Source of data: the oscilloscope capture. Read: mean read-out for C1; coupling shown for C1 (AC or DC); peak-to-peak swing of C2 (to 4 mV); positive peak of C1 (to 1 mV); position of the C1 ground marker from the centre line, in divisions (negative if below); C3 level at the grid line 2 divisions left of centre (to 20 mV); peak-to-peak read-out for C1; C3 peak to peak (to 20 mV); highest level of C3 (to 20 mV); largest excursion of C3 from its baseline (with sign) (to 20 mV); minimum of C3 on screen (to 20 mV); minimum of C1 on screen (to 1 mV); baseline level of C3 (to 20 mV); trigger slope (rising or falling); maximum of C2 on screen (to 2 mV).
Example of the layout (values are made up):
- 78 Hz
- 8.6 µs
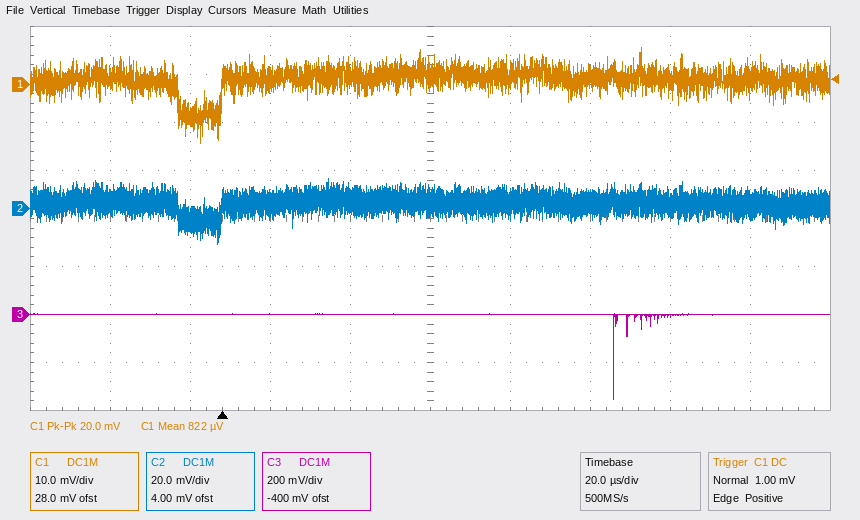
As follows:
- 822 µV
- DC
- 28 mV
- 8 mV
- +2.8 div
- 0 mV
- 20.0 mV
- 360 mV
- 0 mV
- -360 mV
- -360 mV
- -12 mV
- 0 mV
- rising
- 12 mV
